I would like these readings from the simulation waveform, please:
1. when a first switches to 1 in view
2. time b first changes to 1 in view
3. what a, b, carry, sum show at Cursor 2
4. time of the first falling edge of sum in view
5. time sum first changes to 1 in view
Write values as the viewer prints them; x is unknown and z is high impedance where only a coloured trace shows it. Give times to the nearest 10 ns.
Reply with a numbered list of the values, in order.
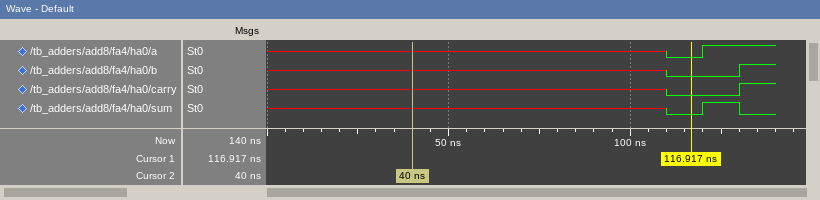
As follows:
1. 120 ns
2. 130 ns
3. a=x, b=x, carry=x, sum=x
4. 130 ns
5. 120 ns
